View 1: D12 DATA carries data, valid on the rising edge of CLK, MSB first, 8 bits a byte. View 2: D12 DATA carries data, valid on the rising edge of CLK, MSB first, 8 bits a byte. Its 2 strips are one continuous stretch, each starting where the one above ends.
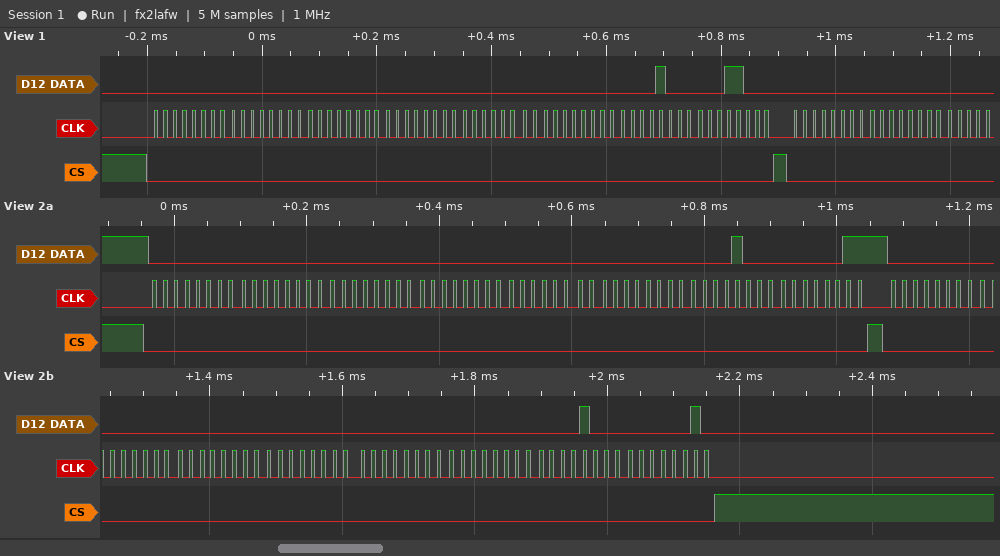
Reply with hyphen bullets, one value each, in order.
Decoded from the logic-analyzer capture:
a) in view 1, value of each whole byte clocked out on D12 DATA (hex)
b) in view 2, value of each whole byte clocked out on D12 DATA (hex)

- 00 00 00 00 00 00 08 18 00 00
- 00 00 00 00 00 00 08 03 00 00 00 00 00 00 08 02
